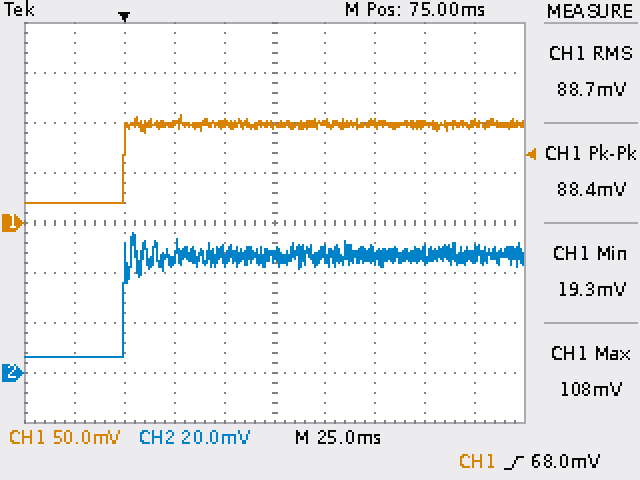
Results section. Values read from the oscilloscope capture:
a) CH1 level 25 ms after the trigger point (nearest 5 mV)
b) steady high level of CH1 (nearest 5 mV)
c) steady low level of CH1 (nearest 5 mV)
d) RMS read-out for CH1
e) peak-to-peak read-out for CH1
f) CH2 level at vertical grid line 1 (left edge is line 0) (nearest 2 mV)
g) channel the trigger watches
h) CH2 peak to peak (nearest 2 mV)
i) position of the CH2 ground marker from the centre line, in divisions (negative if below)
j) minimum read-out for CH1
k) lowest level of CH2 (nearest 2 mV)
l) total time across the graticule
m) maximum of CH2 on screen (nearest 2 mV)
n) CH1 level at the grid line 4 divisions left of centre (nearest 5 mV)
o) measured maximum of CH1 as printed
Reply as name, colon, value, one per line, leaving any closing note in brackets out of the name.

CH1 level 25 ms after the trigger point: 100 mV
steady high level of CH1: 100 mV
steady low level of CH1: 20 mV
RMS read-out for CH1: 88.7 mV
peak-to-peak read-out for CH1: 88.4 mV
CH2 level at vertical grid line 1 (left edge is line 0): 6 mV
channel the trigger watches: CH1
CH2 peak to peak: 50 mV
position of the CH2 ground marker from the centre line, in divisions: -3.0 div
minimum read-out for CH1: 19.3 mV
lowest level of CH2: 6 mV
total time across the graticule: 250 ms
maximum of CH2 on screen: 56 mV
CH1 level at the grid line 4 divisions left of centre: 20 mV
measured maximum of CH1 as printed: 108 mV
